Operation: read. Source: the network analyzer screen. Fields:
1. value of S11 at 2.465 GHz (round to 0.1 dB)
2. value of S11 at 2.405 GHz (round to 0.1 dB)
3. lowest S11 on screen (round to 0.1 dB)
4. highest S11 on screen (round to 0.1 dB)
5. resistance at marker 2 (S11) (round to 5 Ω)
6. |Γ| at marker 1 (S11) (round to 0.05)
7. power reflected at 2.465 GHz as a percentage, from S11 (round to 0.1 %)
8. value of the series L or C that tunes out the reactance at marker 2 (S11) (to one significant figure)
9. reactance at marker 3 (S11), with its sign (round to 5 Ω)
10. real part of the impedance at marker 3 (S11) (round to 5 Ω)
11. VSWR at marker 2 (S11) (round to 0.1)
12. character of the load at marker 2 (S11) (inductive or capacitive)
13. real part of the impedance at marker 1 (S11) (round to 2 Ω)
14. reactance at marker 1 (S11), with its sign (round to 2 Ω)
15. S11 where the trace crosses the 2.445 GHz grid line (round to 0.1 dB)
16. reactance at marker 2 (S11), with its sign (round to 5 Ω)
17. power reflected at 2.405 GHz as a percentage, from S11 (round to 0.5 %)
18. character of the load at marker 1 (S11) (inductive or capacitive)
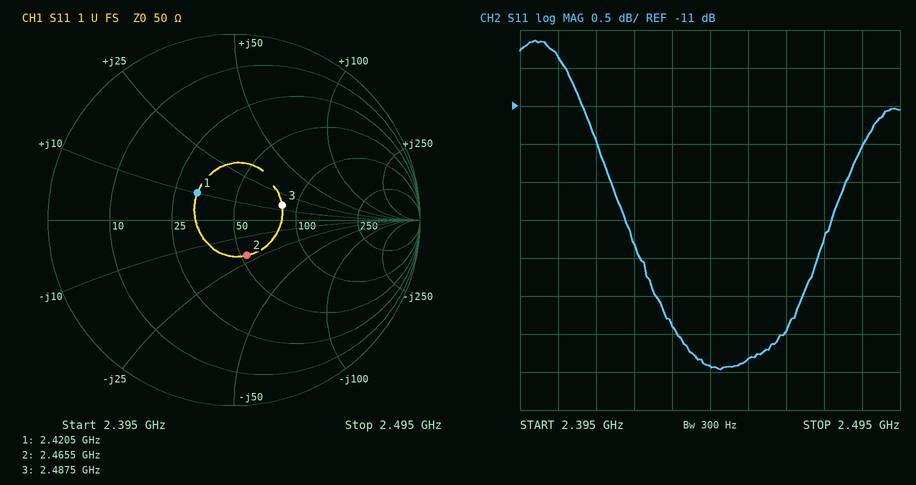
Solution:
-14.0 dB
-10.4 dB
-14.5 dB
-10.1 dB
55 Ω
0.25
4.0 %
1 nH
+15 Ω
85 Ω
1.5
capacitive
32 Ω
+10 Ω
-14.4 dB
-20 Ω
9.0 %
inductive
